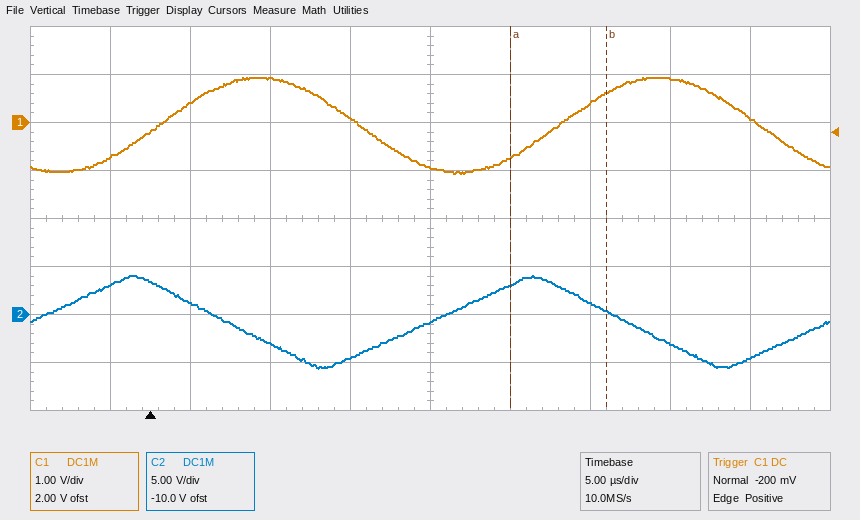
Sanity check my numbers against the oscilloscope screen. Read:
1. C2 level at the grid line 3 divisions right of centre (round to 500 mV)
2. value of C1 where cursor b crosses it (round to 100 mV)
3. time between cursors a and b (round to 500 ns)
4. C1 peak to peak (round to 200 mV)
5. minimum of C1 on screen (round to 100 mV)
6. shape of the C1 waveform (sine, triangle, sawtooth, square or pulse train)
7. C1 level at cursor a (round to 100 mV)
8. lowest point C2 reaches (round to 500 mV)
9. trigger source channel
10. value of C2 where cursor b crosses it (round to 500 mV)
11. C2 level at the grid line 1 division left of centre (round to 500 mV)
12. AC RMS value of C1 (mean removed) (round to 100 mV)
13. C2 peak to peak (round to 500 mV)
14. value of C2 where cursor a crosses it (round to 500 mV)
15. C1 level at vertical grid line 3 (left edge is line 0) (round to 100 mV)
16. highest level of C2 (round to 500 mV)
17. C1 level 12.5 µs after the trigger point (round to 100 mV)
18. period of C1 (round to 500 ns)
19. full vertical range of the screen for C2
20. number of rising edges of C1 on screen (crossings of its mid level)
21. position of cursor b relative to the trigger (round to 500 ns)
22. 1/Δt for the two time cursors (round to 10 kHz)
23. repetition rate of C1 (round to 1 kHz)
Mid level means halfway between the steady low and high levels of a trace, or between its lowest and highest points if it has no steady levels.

-3.0 V
600 mV
6.0 µs
2.0 V
-1.1 V
sine
-700 mV
-5.5 V
C1
500 mV
-4.5 V
700 mV
9.5 V
3.0 V
900 mV
4.0 V
100 mV
25.0 µs
40 V
2
+28.5 µs
170 kHz
40 kHz
